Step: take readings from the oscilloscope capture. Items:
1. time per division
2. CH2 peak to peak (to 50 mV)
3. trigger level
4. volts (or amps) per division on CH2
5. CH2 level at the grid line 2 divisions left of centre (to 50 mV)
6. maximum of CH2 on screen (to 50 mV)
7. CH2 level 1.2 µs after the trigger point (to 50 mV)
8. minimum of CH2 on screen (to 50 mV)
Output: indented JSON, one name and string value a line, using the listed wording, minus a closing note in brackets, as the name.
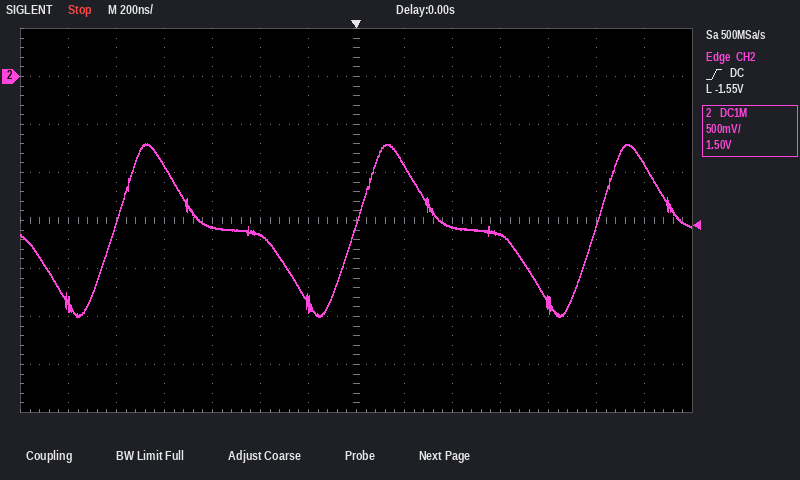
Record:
{
  "time per division": "200 ns",
  "CH2 peak to peak": "1.80 V",
  "trigger level": "-1.55 V",
  "volts (or amps) per division on CH2": "500 mV",
  "CH2 level at the grid line 2 divisions left of centre": "-1.65 V",
  "maximum of CH2 on screen": "-700 mV",
  "CH2 level 1.2 µs after the trigger point": "-900 mV",
  "minimum of CH2 on screen": "-2.50 V"
}
